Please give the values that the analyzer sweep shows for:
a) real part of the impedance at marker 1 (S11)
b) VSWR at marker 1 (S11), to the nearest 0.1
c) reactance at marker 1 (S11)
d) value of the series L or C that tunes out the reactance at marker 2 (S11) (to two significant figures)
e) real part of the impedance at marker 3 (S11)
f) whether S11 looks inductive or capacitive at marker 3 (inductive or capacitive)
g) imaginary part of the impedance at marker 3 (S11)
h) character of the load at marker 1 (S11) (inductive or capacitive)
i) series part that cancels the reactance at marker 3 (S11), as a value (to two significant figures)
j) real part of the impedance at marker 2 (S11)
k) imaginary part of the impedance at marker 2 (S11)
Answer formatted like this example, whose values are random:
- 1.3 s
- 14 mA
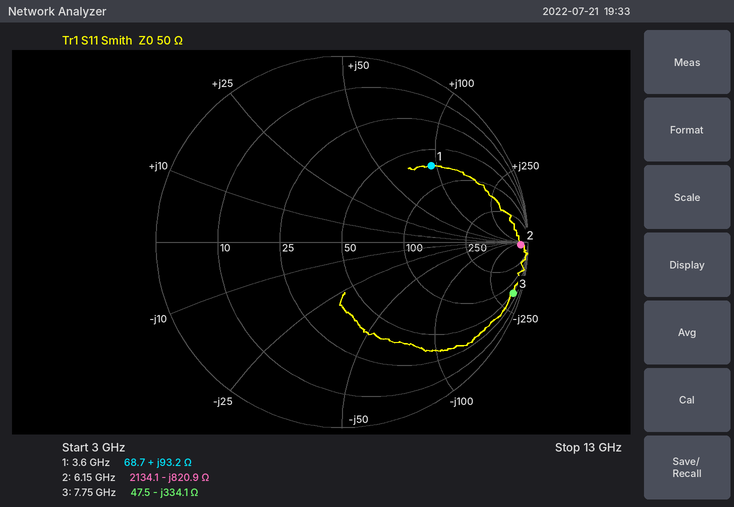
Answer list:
- 68.7 Ω
- 4.4
- +93.2 Ω
- 21 nH
- 47.5 Ω
- capacitive
- -334.1 Ω
- inductive
- 6.9 nH
- 2134.1 Ω
- -820.9 Ω
